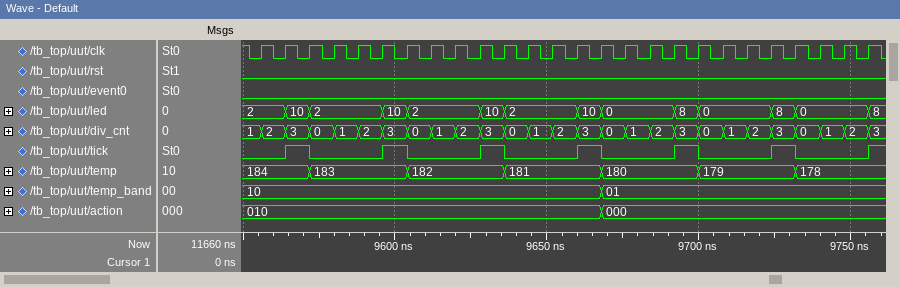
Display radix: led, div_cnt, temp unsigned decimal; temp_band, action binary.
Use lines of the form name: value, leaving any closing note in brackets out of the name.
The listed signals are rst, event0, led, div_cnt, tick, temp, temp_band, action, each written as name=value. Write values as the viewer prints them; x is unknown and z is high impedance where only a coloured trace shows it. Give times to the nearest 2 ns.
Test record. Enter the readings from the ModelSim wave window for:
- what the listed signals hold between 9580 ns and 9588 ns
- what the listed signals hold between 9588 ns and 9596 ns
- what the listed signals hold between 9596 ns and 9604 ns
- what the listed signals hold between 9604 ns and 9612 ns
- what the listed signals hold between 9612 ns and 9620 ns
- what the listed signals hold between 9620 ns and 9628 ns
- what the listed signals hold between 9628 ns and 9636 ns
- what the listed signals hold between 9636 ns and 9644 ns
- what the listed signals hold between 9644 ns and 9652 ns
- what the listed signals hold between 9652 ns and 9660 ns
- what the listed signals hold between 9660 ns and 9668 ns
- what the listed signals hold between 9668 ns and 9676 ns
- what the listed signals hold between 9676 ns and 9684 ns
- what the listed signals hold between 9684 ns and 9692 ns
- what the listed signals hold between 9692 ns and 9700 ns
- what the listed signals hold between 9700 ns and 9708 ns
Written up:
what the listed signals hold between 9580 ns and 9588 ns: rst=0, event0=0, led=2, div_cnt=1, tick=0, temp=183, temp_band=10, action=010
what the listed signals hold between 9588 ns and 9596 ns: rst=0, event0=0, led=2, div_cnt=2, tick=0, temp=183, temp_band=10, action=010
what the listed signals hold between 9596 ns and 9604 ns: rst=0, event0=0, led=10, div_cnt=3, tick=1, temp=183, temp_band=10, action=010
what the listed signals hold between 9604 ns and 9612 ns: rst=0, event0=0, led=2, div_cnt=0, tick=0, temp=182, temp_band=10, action=010
what the listed signals hold between 9612 ns and 9620 ns: rst=0, event0=0, led=2, div_cnt=1, tick=0, temp=182, temp_band=10, action=010
what the listed signals hold between 9620 ns and 9628 ns: rst=0, event0=0, led=2, div_cnt=2, tick=0, temp=182, temp_band=10, action=010
what the listed signals hold between 9628 ns and 9636 ns: rst=0, event0=0, led=10, div_cnt=3, tick=1, temp=182, temp_band=10, action=010
what the listed signals hold between 9636 ns and 9644 ns: rst=0, event0=0, led=2, div_cnt=0, tick=0, temp=181, temp_band=10, action=010
what the listed signals hold between 9644 ns and 9652 ns: rst=0, event0=0, led=2, div_cnt=1, tick=0, temp=181, temp_band=10, action=010
what the listed signals hold between 9652 ns and 9660 ns: rst=0, event0=0, led=2, div_cnt=2, tick=0, temp=181, temp_band=10, action=010
what the listed signals hold between 9660 ns and 9668 ns: rst=0, event0=0, led=10, div_cnt=3, tick=1, temp=181, temp_band=10, action=010
what the listed signals hold between 9668 ns and 9676 ns: rst=0, event0=0, led=0, div_cnt=0, tick=0, temp=180, temp_band=01, action=000
what the listed signals hold between 9676 ns and 9684 ns: rst=0, event0=0, led=0, div_cnt=1, tick=0, temp=180, temp_band=01, action=000
what the listed signals hold between 9684 ns and 9692 ns: rst=0, event0=0, led=0, div_cnt=2, tick=0, temp=180, temp_band=01, action=000
what the listed signals hold between 9692 ns and 9700 ns: rst=0, event0=0, led=8, div_cnt=3, tick=1, temp=180, temp_band=01, action=000
what the listed signals hold between 9700 ns and 9708 ns: rst=0, event0=0, led=0, div_cnt=0, tick=0, temp=179, temp_band=01, action=000
